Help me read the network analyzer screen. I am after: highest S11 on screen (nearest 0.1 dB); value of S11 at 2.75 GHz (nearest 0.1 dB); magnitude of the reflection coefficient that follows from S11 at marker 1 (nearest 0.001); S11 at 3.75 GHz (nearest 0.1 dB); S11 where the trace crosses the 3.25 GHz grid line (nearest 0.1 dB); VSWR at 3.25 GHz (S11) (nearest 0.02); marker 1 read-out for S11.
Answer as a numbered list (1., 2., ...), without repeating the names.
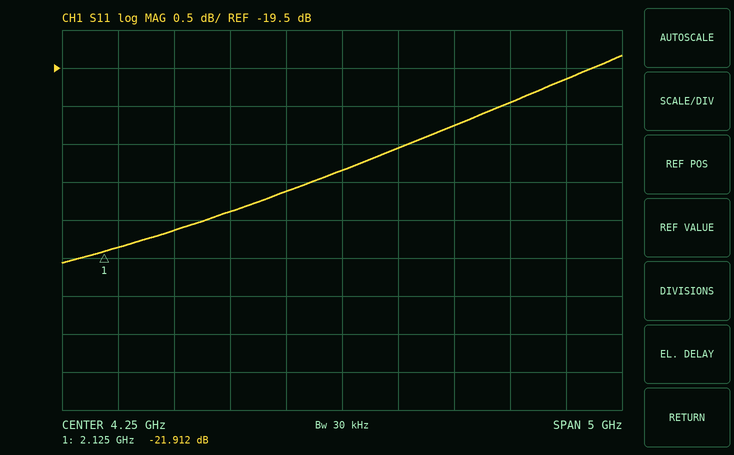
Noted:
1. -19.3 dB
2. -21.6 dB
3. 0.080
4. -21.1 dB
5. -21.4 dB
6. 1.18
7. -21.912 dB
